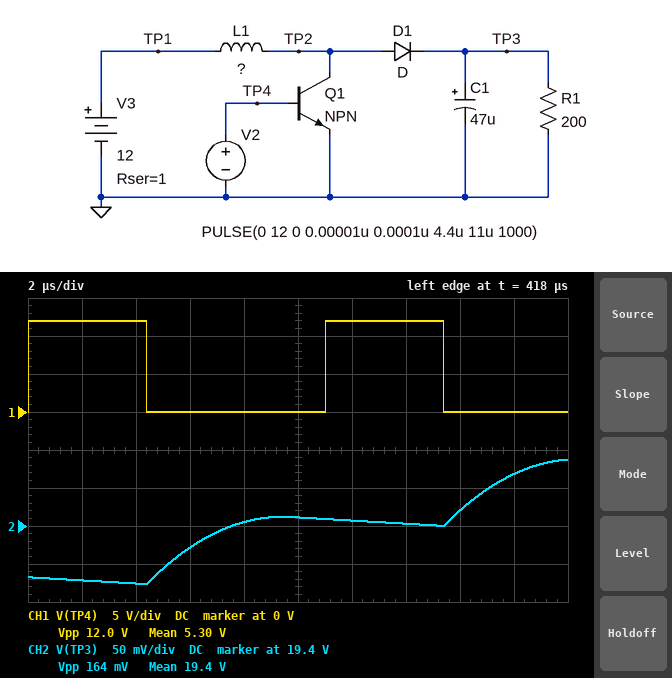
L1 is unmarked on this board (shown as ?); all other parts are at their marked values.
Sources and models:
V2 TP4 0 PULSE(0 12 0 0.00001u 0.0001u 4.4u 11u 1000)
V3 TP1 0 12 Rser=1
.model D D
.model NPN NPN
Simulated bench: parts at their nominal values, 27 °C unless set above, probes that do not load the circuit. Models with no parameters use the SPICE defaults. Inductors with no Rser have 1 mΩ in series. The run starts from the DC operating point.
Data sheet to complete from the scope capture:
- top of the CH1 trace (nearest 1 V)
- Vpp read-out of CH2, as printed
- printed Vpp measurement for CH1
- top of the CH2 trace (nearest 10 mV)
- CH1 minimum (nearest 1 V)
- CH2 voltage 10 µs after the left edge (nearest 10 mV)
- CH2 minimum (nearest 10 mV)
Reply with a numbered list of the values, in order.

1. 12 V
2. 164 mV
3. 12.0 V
4. 19.49 V
5. 0 V
6. 19.41 V
7. 19.32 V
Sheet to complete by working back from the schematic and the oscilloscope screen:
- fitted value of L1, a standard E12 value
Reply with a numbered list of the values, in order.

1. 27 µH
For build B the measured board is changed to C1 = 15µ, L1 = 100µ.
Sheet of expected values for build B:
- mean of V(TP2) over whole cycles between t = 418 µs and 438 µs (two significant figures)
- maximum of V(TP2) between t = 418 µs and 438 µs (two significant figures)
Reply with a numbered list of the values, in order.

1. 12 V
2. 22 V
